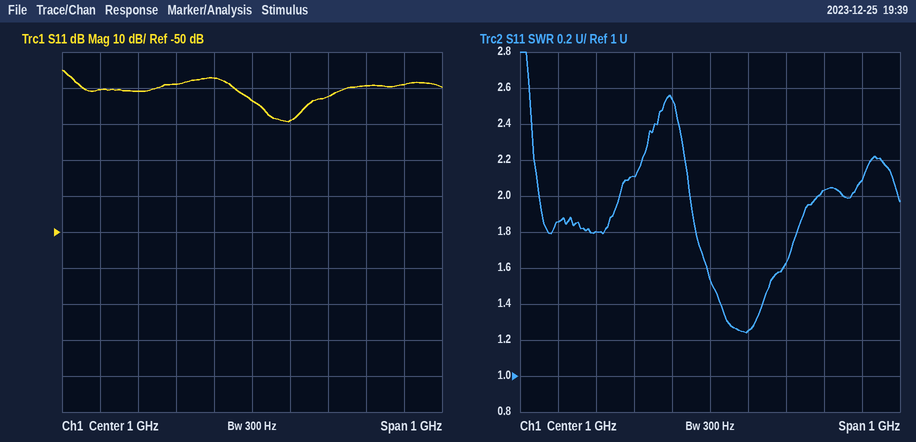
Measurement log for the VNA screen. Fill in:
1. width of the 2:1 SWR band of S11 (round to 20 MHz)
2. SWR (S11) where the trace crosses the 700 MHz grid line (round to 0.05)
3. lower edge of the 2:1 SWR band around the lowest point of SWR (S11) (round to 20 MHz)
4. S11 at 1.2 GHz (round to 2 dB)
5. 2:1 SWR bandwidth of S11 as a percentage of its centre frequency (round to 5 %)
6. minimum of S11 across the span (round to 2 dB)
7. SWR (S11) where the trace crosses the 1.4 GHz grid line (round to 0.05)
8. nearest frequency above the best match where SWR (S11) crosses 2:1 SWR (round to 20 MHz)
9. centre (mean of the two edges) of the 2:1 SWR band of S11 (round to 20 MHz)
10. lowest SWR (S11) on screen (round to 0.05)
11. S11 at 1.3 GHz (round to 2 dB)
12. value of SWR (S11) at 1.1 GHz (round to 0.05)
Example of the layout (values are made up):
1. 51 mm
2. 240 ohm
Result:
1. 340 MHz
2. 1.80
3. 940 MHz
4. -12 dB
5. 30 %
6. -20 dB
7. 2.10
8. 1.28 GHz
9. 1.12 GHz
10. 1.25
11. -10 dB
12. 1.25
